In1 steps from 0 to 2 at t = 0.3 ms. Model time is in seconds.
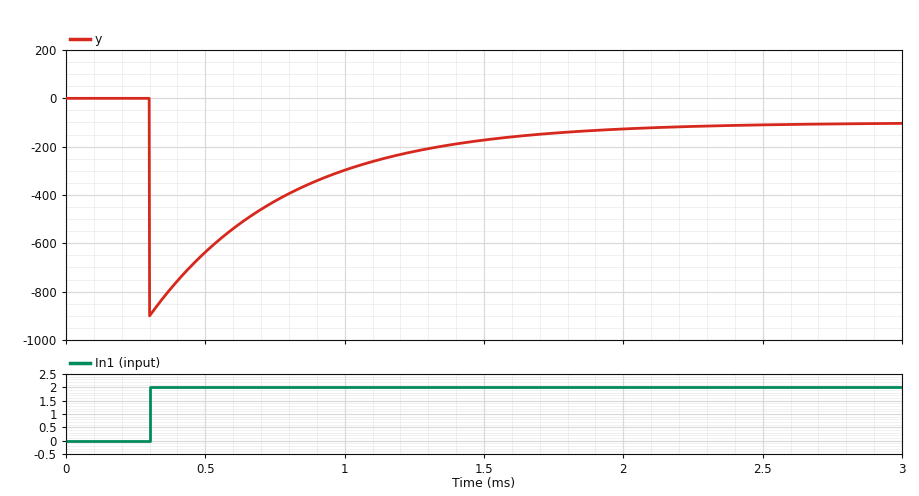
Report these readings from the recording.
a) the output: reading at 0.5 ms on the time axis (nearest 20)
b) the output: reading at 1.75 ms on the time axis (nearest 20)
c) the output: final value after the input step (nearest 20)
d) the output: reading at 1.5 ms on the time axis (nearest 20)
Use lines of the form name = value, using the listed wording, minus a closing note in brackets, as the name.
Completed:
the output: reading at 0.5 ms on the time axis = -640
the output: reading at 1.75 ms on the time axis = -140
the output: final value after the input step = -100
the output: reading at 1.5 ms on the time axis = -180
